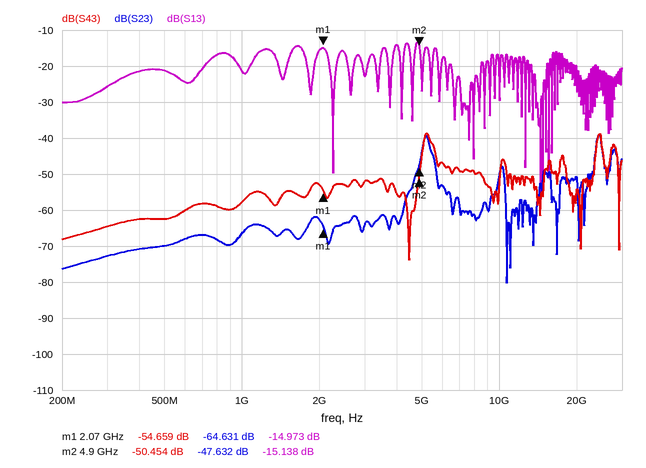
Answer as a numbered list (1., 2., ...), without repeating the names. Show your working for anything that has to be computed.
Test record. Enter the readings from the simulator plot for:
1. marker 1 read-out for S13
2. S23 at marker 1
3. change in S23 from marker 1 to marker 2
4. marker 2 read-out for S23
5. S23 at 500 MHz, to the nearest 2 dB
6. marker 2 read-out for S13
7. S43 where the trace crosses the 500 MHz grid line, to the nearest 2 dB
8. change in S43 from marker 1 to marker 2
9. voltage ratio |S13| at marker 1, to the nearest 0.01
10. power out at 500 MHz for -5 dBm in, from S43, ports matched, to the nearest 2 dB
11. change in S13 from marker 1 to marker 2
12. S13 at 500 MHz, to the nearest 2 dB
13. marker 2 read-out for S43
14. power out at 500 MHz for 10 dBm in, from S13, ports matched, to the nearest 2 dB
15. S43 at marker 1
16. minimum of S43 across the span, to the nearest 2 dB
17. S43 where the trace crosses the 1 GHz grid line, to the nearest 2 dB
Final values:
1. -14.973 dB
2. -64.631 dB
3. -47.632 − (-64.631) = 16.999 dB
4. -47.632 dB
5. -70 dB
6. -15.138 dB
7. -62 dB
8. -50.454 − (-54.659) = 4.205 dB
9. 10^(-14.973/20) ≈ 0.18
10. -5 dBm + (-62 dB) = -68 dBm
11. -15.138 − (-14.973) = -0.165 dB
12. -22 dB
13. -50.454 dB
14. 10 dBm + (-22 dB) = -12 dBm
15. -54.659 dB
16. -74 dB
17. -58 dB
